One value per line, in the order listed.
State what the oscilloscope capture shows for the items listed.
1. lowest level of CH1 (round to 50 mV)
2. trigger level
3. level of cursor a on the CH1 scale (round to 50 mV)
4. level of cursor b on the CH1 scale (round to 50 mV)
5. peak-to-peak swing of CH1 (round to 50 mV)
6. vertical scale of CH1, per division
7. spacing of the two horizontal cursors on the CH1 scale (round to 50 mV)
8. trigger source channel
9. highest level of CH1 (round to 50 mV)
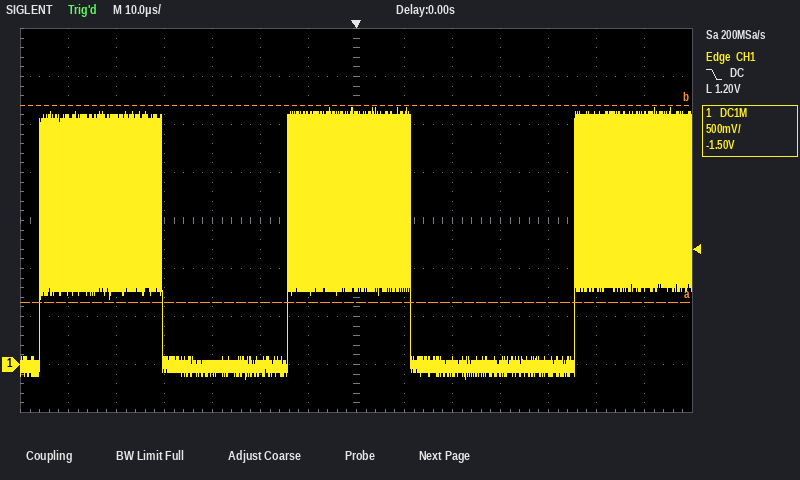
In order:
-150 mV
1.20 V
650 mV
2.70 V
2.85 V
500 mV
2.05 V
CH1
2.70 V
